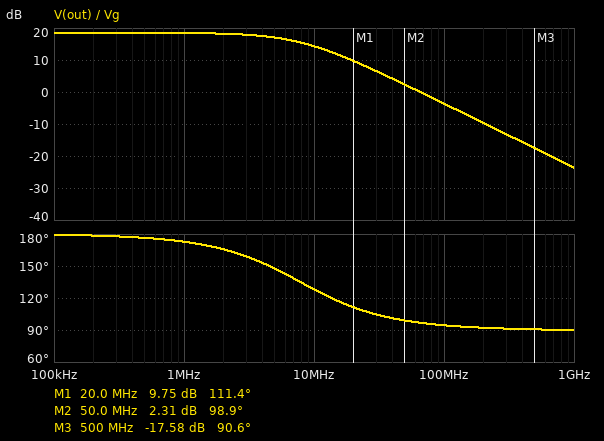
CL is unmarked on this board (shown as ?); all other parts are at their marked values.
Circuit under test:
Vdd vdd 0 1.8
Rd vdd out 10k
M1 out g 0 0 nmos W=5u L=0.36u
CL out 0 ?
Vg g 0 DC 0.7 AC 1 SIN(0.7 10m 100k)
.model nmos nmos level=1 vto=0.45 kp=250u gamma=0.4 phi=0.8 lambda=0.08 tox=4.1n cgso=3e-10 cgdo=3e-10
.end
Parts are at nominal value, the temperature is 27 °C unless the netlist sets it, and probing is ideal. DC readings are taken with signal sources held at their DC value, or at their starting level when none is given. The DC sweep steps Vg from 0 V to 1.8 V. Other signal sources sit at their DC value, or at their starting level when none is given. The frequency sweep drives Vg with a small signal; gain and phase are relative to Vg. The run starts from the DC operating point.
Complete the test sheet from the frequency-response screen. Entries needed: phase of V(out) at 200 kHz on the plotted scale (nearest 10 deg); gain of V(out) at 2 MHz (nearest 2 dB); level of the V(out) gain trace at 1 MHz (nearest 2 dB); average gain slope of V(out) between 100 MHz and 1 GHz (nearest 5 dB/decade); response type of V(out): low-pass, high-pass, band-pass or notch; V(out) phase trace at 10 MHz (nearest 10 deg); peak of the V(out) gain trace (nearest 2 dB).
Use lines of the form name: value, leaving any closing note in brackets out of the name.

phase of V(out) at 200 kHz on the plotted scale: 180 deg
gain of V(out) at 2 MHz: 18 dB
level of the V(out) gain trace at 1 MHz: 18 dB
average gain slope of V(out) between 100 MHz and 1 GHz: -20 dB/decade
response type of V(out): low-pass, high-pass, band-pass or notch: low-pass
V(out) phase trace at 10 MHz: 130 deg
peak of the V(out) gain trace: 18 dB
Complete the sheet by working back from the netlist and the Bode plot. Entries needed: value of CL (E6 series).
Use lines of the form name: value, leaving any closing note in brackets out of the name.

value of CL: 2.2 pF
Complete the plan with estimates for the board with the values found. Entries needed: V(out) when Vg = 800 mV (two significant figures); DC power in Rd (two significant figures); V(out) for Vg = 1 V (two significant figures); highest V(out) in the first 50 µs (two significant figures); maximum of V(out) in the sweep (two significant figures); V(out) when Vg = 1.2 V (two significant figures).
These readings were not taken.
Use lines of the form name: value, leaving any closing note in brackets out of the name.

V(out) when Vg = 800 mV: 180 mV
DC power in Rd: 130 µW
V(out) for Vg = 1 V: 97 mV
highest V(out) in the first 50 µs: 740 mV
maximum of V(out) in the sweep: 1.8 V
V(out) when Vg = 1.2 V: 69 mV
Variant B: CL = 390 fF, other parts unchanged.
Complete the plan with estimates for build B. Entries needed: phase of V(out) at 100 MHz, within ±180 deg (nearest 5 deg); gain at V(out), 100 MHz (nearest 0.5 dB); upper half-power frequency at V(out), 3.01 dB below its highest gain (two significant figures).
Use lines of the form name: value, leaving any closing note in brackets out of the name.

phase of V(out) at 100 MHz, within ±180 deg: 115 deg
gain at V(out), 100 MHz: 10.5 dB
upper half-power frequency at V(out), 3.01 dB below its highest gain: 44 MHz
